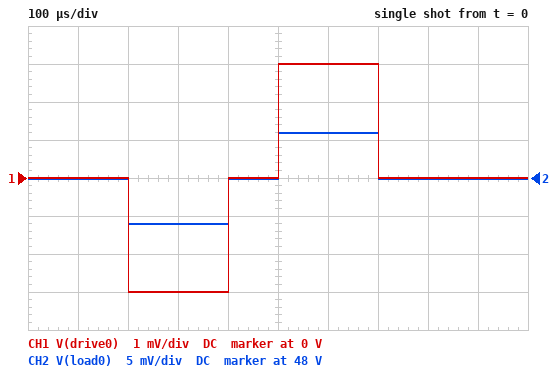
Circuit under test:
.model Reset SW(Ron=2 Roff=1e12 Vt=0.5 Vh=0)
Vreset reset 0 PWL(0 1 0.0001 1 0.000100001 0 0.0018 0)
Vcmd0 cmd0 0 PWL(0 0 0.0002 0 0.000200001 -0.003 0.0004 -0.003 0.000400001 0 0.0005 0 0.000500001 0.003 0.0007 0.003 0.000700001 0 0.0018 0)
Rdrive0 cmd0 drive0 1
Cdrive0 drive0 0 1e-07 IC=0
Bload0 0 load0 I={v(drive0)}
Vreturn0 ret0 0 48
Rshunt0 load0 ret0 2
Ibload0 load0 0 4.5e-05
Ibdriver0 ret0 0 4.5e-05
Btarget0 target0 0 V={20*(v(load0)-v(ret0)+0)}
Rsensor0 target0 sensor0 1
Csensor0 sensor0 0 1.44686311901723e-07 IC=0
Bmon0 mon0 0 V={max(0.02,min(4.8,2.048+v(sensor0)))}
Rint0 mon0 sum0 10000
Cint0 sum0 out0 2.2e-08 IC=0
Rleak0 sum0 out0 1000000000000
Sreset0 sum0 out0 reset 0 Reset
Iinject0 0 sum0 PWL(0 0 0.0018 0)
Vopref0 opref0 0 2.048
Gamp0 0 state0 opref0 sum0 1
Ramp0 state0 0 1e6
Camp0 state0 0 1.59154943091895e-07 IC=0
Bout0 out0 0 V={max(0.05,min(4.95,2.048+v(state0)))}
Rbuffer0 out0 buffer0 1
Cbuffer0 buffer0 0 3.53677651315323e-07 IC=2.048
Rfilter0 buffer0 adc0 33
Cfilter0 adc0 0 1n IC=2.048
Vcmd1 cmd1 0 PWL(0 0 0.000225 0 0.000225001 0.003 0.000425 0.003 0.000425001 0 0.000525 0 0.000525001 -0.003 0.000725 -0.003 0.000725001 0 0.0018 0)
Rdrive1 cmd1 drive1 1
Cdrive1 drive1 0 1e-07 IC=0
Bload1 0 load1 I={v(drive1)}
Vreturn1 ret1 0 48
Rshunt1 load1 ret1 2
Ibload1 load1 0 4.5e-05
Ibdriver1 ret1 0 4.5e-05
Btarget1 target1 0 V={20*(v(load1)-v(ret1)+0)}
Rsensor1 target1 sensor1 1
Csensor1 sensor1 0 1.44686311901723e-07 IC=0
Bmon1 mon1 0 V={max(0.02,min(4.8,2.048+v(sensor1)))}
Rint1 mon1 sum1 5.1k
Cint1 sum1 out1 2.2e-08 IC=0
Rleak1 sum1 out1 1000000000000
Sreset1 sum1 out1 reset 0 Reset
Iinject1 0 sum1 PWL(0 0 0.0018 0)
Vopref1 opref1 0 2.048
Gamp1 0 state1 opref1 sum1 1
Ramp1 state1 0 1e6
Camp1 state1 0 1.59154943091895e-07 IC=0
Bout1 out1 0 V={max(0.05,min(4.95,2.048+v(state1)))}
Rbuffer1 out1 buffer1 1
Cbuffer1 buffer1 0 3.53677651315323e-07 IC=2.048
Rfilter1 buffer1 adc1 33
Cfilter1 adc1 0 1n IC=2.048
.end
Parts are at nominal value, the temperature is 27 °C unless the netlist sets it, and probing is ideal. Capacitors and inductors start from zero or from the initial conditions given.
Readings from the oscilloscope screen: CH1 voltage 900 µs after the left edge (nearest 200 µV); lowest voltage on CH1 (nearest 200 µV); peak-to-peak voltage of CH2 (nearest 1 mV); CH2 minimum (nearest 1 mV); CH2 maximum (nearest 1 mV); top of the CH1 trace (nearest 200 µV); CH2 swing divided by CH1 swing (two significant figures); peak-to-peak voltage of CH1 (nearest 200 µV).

0 V
-3.0 mV
12 mV
47.994 V
48.006 V
3.0 mV
2.0
6.0 mV
